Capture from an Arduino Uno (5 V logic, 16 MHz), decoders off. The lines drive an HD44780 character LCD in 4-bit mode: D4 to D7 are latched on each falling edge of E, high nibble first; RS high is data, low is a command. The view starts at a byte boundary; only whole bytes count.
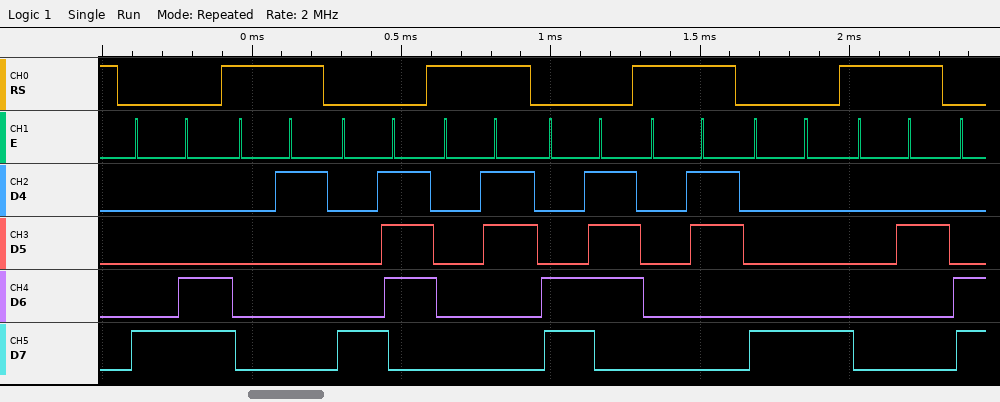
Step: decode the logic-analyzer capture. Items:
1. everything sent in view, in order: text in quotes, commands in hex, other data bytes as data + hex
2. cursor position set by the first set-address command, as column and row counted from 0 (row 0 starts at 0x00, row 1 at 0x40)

0x8C data 01 0x87 data 03 0xC7 data 03 0x88 data 02
column 12, row 0
